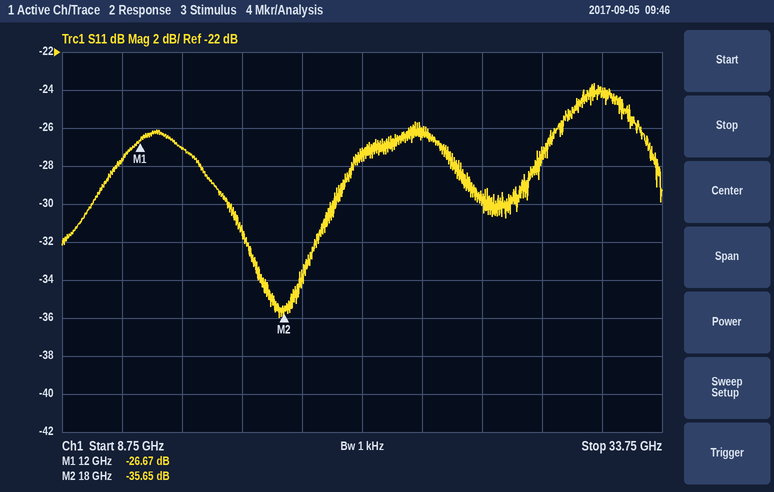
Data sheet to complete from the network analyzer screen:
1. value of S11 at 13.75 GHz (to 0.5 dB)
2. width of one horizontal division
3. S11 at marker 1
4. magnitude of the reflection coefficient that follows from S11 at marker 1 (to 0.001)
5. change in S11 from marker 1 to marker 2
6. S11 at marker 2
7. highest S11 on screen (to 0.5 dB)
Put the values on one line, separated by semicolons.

-27.0 dB; 2.5 GHz; -26.67 dB; 0.046; -8.98 dB; -35.65 dB; -23.5 dB
